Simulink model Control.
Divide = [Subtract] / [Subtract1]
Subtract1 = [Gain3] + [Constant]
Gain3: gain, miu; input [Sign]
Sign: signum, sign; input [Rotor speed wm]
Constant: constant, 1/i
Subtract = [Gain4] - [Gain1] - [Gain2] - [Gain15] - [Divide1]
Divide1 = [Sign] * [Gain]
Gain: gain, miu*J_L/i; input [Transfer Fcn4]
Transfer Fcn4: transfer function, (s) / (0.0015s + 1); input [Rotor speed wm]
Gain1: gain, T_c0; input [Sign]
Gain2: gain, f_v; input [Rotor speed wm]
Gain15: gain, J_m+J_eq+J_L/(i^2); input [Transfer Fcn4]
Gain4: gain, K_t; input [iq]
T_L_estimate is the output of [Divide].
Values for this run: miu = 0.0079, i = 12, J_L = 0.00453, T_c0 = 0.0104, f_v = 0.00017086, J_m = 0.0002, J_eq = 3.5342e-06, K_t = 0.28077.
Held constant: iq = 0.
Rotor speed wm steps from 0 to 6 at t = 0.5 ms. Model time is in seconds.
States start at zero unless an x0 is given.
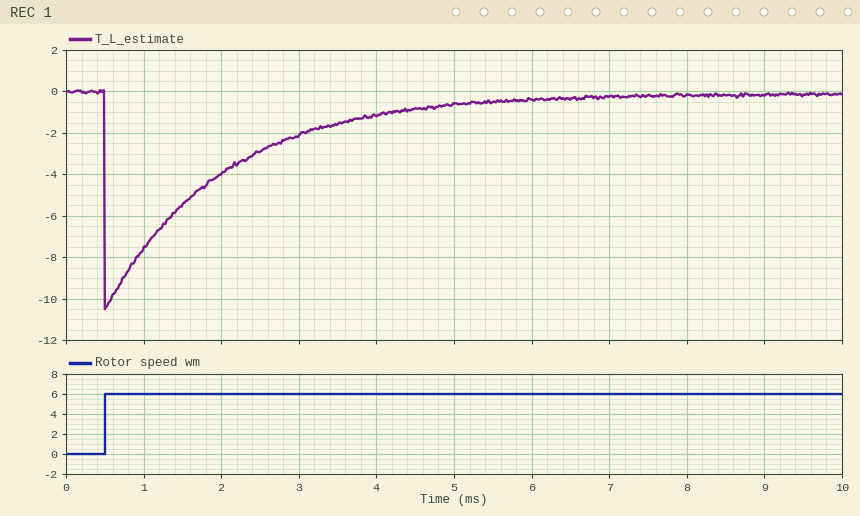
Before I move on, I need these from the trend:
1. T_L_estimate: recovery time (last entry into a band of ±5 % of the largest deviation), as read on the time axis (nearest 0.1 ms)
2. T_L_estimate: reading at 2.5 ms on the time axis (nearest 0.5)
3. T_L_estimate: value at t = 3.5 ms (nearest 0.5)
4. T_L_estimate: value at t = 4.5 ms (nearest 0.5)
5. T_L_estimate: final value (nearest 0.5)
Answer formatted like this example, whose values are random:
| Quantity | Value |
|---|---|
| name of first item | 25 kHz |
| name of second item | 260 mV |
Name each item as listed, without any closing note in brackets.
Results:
| Quantity | Value |
|---|---|
| T_L_estimate: recovery time (last entry into a band of ±5 % of the largest deviation), as read on the time axis | 5.0 ms |
| T_L_estimate: reading at 2.5 ms on the time axis | -3.0 |
| T_L_estimate: value at t = 3.5 ms | -1.5 |
| T_L_estimate: value at t = 4.5 ms | -1.0 |
| T_L_estimate: final value | 0.0 |
